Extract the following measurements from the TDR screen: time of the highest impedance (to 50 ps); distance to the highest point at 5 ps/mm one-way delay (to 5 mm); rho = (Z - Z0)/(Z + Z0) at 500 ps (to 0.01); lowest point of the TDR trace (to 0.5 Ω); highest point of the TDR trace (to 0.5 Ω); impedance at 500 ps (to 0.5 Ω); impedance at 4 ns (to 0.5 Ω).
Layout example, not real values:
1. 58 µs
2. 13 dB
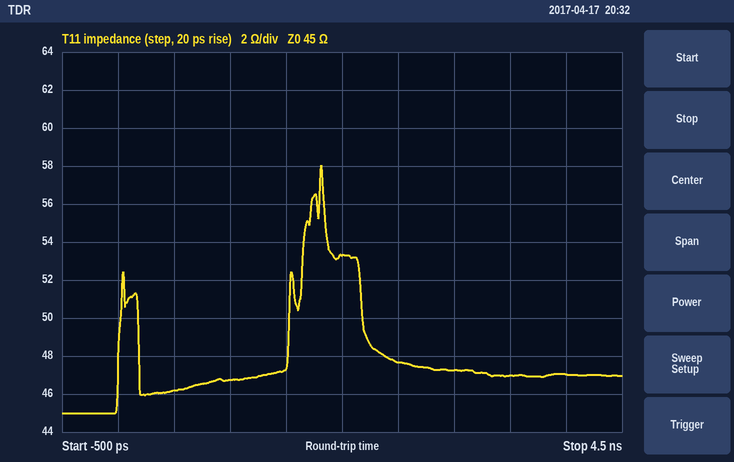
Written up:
1. 1.80 ns
2. 180 mm
3. +0.01
4. 45.0 Ω
5. 58.0 Ω
6. 46.0 Ω
7. 47.0 Ω
